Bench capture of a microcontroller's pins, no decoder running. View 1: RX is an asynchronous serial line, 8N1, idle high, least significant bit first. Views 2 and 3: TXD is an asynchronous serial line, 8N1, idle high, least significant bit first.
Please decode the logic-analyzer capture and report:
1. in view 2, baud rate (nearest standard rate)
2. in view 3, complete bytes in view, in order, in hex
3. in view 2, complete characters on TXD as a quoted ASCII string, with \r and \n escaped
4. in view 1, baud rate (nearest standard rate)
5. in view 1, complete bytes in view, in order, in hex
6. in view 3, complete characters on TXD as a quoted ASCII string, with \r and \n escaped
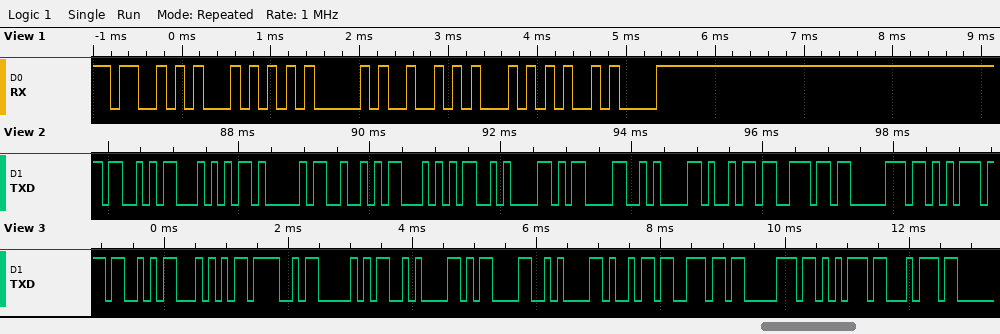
9600 baud
53 54 4F 50 0A 0D 0A 69 6E 70 75 74
"START\n\r\ninpu"
9600 baud
53 54 41 52 54 0A
"STOP\n\r\ninput"
